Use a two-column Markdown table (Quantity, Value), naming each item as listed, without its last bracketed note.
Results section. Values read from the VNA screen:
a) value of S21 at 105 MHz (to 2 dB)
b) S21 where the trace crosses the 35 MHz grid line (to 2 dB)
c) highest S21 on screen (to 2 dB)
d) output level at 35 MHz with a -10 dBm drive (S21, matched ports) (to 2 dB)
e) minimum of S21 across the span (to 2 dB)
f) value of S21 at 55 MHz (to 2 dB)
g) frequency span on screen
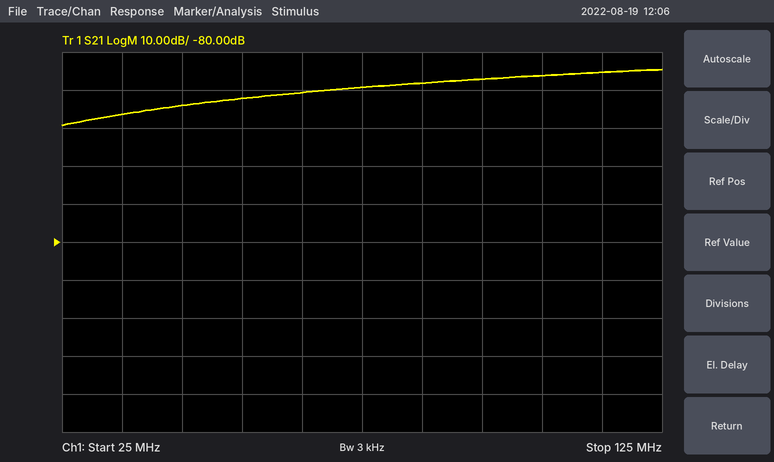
| Quantity | Value |
|---|---|
| value of S21 at 105 MHz | -36 dB |
| S21 where the trace crosses the 35 MHz grid line | -46 dB |
| highest S21 on screen | -34 dB |
| output level at 35 MHz with a -10 dBm drive (S21, matched ports) | -56 dBm |
| minimum of S21 across the span | -50 dB |
| value of S21 at 55 MHz | -42 dB |
| frequency span on screen | 100 MHz |
